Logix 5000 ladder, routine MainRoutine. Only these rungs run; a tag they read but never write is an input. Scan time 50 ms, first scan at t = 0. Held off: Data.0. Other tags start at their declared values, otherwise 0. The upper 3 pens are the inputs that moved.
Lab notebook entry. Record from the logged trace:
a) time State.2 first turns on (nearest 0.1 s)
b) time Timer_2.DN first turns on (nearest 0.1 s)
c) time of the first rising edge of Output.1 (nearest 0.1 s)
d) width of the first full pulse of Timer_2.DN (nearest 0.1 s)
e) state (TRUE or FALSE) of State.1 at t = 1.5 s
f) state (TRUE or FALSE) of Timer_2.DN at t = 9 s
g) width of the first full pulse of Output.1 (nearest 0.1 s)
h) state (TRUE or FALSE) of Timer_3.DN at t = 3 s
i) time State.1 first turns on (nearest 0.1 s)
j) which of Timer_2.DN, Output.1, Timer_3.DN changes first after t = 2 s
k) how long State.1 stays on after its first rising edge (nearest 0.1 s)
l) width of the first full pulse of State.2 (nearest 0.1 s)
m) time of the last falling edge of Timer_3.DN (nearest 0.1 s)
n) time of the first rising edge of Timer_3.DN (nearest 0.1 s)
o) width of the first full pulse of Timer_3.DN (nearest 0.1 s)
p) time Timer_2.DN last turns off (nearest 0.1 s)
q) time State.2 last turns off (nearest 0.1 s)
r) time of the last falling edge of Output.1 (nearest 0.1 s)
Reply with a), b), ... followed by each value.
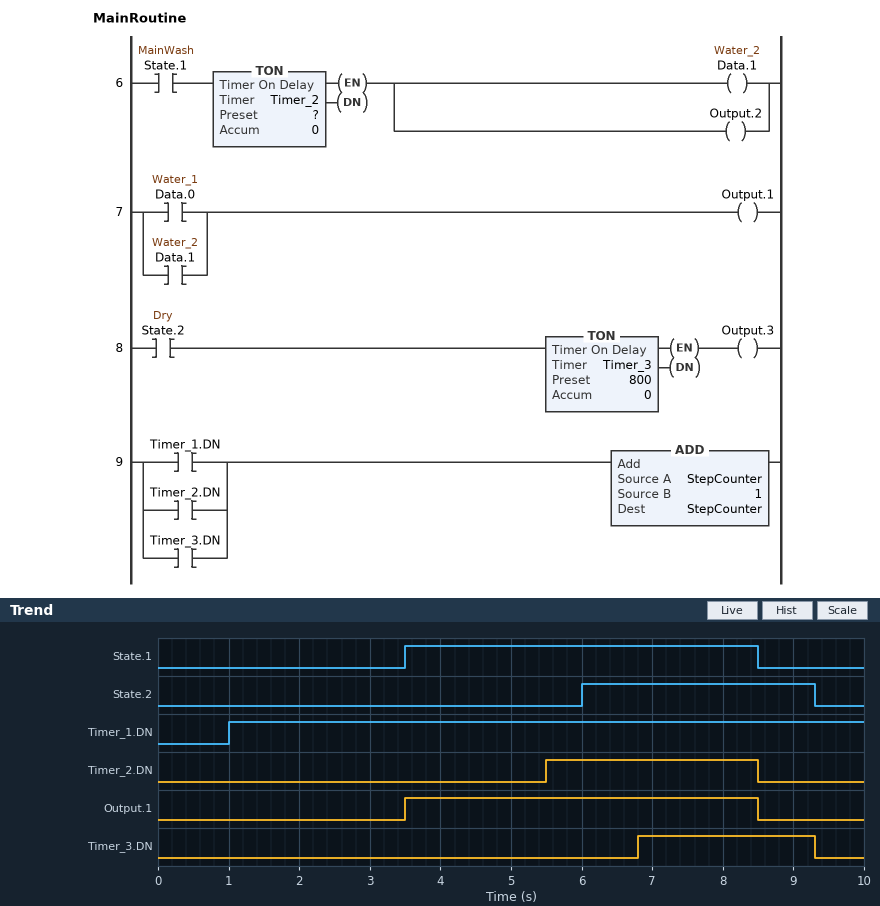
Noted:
a) 6.0 s
b) 5.5 s
c) 3.5 s
d) 3.0 s
e) FALSE
f) FALSE
g) 5.0 s
h) FALSE
i) 3.5 s
j) Output.1
k) 5.0 s
l) 3.3 s
m) 9.3 s
n) 6.8 s
o) 2.5 s
p) 8.5 s
q) 9.3 s
r) 8.5 s
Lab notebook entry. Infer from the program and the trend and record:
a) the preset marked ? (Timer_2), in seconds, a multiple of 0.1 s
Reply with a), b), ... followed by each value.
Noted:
a) 2.0 s
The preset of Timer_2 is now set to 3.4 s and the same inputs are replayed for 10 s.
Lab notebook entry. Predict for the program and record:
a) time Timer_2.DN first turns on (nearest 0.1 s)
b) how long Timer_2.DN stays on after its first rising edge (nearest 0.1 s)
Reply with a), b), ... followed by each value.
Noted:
a) 6.9 s
b) 1.6 s
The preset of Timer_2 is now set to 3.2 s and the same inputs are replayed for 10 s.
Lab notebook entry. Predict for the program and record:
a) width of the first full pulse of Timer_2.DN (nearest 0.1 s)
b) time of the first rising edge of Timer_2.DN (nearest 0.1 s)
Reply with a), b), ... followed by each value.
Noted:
a) 1.8 s
b) 6.7 s
